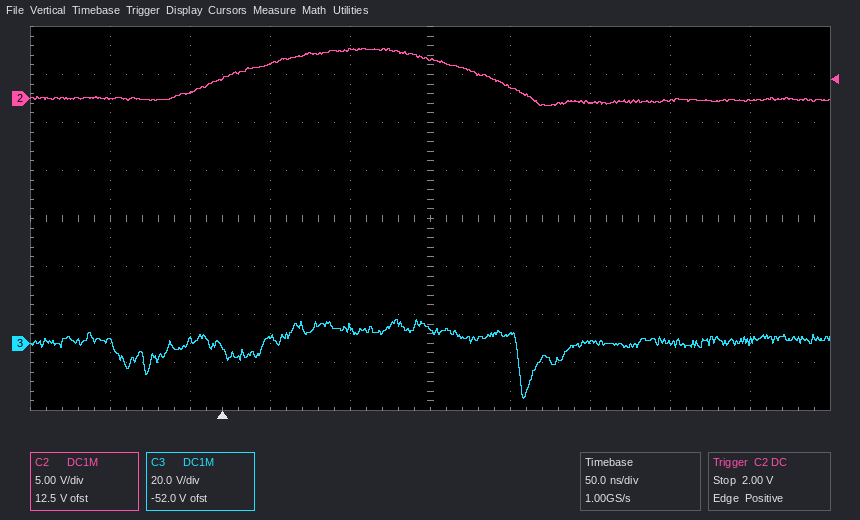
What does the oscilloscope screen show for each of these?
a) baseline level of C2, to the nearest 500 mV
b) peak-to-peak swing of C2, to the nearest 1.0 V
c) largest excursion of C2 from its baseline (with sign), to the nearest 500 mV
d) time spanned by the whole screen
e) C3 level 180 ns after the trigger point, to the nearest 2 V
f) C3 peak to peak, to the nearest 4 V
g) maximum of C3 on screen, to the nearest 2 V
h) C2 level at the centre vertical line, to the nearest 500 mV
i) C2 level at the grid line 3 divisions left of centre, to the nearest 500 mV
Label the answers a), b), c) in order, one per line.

a) 0.0 V
b) 6.0 V
c) +5.5 V
d) 500 ns
e) 4 V
f) 32 V
g) 10 V
h) 4.0 V
i) 500 mV
